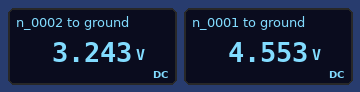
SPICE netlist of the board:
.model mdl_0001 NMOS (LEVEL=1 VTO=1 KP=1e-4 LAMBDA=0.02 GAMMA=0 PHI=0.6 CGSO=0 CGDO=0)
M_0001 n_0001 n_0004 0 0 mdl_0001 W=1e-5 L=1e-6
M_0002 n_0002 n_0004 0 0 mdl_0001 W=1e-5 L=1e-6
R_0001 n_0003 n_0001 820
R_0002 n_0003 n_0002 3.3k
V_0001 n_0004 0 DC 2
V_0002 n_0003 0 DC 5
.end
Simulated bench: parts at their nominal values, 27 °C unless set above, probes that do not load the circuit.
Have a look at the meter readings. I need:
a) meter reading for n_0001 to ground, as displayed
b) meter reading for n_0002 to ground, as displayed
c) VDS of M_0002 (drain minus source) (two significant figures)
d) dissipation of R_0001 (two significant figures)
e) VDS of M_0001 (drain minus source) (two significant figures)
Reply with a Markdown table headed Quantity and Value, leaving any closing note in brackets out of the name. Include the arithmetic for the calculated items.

| Quantity | Value |
|---|---|
| meter reading for n_0001 to ground, as displayed | 4.553 V |
| meter reading for n_0002 to ground, as displayed | 3.243 V |
| VDS of M_0002 (drain minus source) | 3.243 V = 3.2 V |
| dissipation of R_0001 | (5 V - 4.553 V)^2 / 820 Ω = 240 µW |
| VDS of M_0001 (drain minus source) | 4.553 V = 4.6 V |
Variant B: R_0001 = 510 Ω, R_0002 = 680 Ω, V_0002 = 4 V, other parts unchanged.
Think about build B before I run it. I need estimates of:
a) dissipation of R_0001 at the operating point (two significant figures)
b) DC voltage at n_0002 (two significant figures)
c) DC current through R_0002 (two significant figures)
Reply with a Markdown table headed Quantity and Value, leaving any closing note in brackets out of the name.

| Quantity | Value |
|---|---|
| dissipation of R_0001 at the operating point | 150 µW |
| DC voltage at n_0002 | 3.6 V |
| DC current through R_0002 | 540 µA |
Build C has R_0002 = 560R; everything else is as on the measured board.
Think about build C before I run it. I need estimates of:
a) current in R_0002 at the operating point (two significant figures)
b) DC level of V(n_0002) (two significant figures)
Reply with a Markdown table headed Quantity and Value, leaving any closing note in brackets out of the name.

| Quantity | Value |
|---|---|
| current in R_0002 at the operating point | 550 µA |
| DC level of V(n_0002) | 4.7 V |
